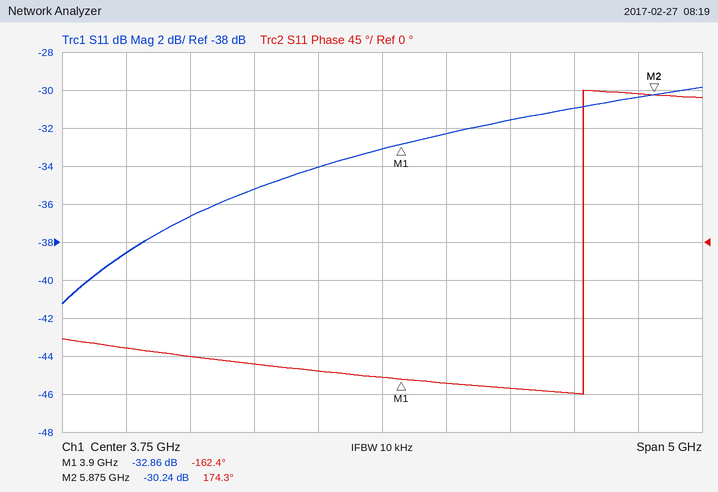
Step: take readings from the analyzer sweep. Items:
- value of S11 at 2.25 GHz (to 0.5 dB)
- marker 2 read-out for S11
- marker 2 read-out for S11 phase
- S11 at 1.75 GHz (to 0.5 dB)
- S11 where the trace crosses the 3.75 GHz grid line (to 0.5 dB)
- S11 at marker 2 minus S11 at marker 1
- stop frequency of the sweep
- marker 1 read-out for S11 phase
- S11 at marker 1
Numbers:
-36.5 dB
-30.24 dB
174.3°
-38.5 dB
-33.0 dB
2.62 dB
6.25 GHz
-162.4°
-32.86 dB
